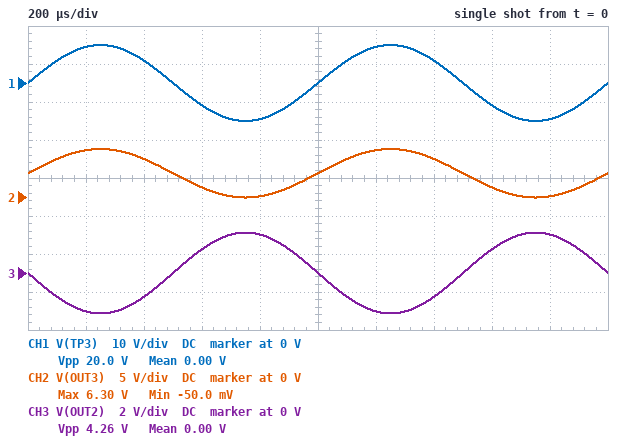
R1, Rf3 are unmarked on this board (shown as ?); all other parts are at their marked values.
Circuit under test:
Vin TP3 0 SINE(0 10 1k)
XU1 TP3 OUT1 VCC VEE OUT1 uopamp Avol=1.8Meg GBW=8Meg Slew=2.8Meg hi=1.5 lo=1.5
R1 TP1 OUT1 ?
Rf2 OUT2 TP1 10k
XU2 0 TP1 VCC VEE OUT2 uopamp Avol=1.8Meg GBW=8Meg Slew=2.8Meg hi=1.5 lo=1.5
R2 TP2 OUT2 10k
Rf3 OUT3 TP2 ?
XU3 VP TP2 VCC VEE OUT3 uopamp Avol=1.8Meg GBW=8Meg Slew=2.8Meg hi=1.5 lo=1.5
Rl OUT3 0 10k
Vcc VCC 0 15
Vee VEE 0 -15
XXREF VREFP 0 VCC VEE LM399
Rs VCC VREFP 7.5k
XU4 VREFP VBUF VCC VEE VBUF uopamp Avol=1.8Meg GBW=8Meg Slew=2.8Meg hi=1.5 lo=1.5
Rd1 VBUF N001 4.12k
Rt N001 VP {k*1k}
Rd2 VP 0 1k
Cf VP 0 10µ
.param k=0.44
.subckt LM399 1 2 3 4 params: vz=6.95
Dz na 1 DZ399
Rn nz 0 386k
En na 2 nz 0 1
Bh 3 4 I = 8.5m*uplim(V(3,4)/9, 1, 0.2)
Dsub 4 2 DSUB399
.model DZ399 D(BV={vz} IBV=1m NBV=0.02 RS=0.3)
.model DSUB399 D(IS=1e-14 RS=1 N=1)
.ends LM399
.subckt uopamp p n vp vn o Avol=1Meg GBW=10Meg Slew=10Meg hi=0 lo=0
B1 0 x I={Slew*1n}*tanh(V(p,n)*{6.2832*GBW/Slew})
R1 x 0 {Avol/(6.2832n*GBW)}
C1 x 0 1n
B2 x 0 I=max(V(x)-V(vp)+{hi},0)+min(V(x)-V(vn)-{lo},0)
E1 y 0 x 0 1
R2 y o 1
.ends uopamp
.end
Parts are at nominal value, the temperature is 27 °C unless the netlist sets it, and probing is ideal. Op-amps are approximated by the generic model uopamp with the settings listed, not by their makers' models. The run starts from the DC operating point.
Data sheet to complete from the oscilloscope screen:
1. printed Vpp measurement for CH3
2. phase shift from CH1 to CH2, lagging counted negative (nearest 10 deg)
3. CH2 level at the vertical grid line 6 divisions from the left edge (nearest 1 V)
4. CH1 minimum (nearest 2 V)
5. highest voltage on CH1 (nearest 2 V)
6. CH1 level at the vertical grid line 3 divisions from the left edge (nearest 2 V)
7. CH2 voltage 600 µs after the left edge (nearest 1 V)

4.26 V
0 deg
6 V
-10 V
10 V
-6 V
1 V
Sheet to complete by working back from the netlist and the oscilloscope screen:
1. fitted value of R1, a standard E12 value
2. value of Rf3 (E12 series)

47 kΩ
15 kΩ
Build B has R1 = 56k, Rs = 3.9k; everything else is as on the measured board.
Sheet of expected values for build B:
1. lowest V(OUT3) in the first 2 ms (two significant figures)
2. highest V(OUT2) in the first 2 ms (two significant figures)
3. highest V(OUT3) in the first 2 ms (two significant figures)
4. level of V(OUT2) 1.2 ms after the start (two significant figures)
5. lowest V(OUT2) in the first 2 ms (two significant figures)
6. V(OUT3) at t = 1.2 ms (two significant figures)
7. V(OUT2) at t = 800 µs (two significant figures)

450 mV
1.8 V
5.8 V
-1.7 V
-1.8 V
5.7 V
1.7 V
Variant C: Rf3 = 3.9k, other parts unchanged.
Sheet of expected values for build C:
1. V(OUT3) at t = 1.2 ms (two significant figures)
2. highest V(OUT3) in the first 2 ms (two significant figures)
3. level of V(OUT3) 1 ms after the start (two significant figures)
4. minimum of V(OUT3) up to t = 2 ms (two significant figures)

2.5 V
2.6 V
1.7 V
910 mV
